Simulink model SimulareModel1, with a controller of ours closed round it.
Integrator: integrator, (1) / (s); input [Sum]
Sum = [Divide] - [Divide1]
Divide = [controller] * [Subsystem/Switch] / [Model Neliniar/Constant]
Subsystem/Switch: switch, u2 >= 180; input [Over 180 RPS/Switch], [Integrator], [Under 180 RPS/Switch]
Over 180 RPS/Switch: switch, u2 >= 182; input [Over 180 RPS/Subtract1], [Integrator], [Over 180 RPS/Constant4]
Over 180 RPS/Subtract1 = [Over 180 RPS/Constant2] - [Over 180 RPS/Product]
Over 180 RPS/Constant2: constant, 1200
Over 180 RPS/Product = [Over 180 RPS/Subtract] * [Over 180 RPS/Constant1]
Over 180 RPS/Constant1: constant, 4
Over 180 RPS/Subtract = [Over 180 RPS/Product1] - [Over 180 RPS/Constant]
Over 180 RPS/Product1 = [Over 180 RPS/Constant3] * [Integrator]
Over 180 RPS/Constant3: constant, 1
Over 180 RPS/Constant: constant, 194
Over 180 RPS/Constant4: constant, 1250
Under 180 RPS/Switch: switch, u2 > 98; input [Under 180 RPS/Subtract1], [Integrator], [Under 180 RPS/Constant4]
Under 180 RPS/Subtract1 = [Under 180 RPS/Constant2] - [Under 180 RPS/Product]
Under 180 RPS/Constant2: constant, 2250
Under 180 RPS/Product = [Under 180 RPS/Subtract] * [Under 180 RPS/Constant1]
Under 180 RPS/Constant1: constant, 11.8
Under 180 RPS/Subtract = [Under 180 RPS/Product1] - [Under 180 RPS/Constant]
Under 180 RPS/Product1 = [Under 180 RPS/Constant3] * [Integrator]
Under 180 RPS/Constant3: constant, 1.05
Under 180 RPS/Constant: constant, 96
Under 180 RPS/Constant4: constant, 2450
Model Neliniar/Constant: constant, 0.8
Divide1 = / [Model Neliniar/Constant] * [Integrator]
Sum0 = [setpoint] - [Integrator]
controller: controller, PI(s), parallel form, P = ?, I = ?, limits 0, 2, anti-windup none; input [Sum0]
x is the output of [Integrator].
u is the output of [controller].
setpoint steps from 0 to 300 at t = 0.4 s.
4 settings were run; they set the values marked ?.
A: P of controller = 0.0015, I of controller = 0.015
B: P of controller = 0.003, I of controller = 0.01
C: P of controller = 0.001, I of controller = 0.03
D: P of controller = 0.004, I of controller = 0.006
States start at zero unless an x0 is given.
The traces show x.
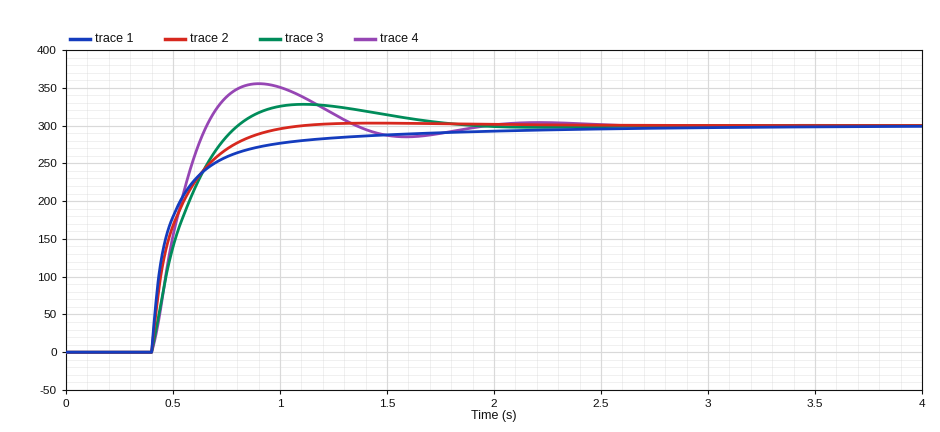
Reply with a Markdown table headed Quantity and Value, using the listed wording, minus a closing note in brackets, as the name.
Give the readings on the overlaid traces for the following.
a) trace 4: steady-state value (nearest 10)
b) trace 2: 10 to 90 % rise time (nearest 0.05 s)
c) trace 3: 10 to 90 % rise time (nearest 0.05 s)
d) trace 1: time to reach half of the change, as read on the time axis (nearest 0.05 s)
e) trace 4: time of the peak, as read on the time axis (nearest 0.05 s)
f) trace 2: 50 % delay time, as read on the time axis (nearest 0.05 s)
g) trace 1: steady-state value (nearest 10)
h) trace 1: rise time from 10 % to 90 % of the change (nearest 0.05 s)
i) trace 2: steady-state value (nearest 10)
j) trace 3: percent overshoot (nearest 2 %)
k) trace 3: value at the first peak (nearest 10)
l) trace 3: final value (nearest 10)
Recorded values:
| Quantity | Value |
|---|---|
| trace 4: steady-state value | 300 |
| trace 2: 10 to 90 % rise time | 0.35 s |
| trace 3: 10 to 90 % rise time | 0.30 s |
| trace 1: time to reach half of the change, as read on the time axis | 0.45 s |
| trace 4: time of the peak, as read on the time axis | 0.90 s |
| trace 2: 50 % delay time, as read on the time axis | 0.50 s |
| trace 1: steady-state value | 300 |
| trace 1: rise time from 10 % to 90 % of the change | 0.45 s |
| trace 2: steady-state value | 300 |
| trace 3: percent overshoot | 10 % |
| trace 3: value at the first peak | 330 |
| trace 3: final value | 300 |
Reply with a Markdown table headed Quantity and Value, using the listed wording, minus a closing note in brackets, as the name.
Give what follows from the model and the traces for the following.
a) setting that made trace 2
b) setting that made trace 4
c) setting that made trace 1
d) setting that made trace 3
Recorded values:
| Quantity | Value |
|---|---|
| setting that made trace 2 | B |
| setting that made trace 4 | C |
| setting that made trace 1 | D |
| setting that made trace 3 | A |
